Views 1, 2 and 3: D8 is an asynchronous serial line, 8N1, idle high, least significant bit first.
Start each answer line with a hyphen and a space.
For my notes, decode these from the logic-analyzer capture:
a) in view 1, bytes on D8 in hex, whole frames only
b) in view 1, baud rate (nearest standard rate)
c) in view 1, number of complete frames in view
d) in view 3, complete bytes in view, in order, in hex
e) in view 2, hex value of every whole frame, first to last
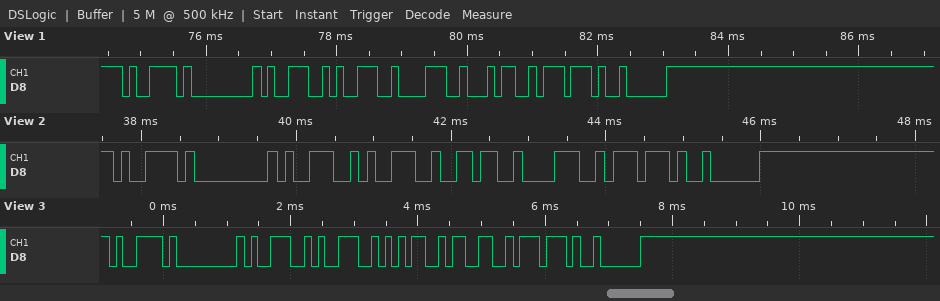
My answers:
- 79 00 39 39 38 34 77 02
- 9600 baud
- 8
- 79 00 39 39 35 33 77 02
- 79 00 39 39 36 38 77 02
